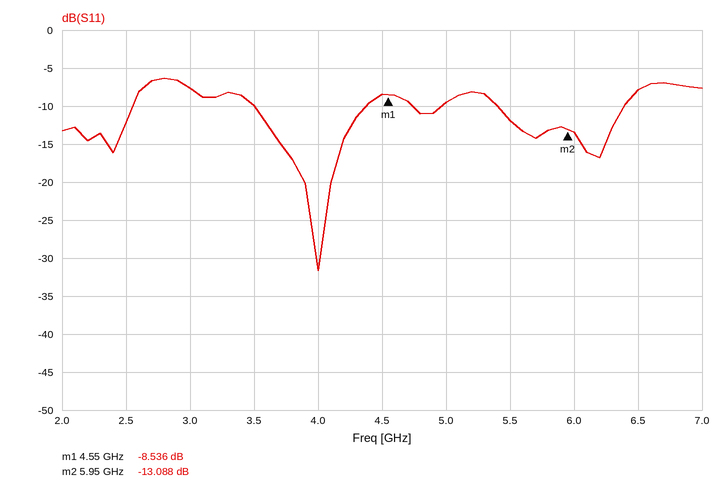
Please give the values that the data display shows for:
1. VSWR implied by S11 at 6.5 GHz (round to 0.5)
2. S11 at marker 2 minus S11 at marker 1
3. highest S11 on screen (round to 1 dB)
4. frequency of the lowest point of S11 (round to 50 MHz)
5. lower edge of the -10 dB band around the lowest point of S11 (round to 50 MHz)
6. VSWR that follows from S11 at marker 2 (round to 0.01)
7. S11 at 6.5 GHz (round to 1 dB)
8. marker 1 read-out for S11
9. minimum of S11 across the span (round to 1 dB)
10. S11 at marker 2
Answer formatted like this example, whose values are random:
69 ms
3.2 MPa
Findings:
2.5
-4.552 dB
-6 dB
4.00 GHz
3.50 GHz
1.57
-8 dB
-8.536 dB
-32 dB
-13.088 dB
